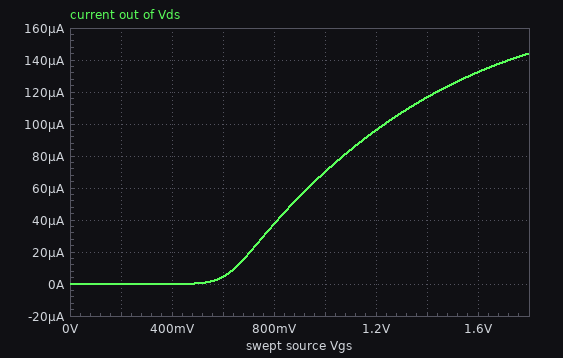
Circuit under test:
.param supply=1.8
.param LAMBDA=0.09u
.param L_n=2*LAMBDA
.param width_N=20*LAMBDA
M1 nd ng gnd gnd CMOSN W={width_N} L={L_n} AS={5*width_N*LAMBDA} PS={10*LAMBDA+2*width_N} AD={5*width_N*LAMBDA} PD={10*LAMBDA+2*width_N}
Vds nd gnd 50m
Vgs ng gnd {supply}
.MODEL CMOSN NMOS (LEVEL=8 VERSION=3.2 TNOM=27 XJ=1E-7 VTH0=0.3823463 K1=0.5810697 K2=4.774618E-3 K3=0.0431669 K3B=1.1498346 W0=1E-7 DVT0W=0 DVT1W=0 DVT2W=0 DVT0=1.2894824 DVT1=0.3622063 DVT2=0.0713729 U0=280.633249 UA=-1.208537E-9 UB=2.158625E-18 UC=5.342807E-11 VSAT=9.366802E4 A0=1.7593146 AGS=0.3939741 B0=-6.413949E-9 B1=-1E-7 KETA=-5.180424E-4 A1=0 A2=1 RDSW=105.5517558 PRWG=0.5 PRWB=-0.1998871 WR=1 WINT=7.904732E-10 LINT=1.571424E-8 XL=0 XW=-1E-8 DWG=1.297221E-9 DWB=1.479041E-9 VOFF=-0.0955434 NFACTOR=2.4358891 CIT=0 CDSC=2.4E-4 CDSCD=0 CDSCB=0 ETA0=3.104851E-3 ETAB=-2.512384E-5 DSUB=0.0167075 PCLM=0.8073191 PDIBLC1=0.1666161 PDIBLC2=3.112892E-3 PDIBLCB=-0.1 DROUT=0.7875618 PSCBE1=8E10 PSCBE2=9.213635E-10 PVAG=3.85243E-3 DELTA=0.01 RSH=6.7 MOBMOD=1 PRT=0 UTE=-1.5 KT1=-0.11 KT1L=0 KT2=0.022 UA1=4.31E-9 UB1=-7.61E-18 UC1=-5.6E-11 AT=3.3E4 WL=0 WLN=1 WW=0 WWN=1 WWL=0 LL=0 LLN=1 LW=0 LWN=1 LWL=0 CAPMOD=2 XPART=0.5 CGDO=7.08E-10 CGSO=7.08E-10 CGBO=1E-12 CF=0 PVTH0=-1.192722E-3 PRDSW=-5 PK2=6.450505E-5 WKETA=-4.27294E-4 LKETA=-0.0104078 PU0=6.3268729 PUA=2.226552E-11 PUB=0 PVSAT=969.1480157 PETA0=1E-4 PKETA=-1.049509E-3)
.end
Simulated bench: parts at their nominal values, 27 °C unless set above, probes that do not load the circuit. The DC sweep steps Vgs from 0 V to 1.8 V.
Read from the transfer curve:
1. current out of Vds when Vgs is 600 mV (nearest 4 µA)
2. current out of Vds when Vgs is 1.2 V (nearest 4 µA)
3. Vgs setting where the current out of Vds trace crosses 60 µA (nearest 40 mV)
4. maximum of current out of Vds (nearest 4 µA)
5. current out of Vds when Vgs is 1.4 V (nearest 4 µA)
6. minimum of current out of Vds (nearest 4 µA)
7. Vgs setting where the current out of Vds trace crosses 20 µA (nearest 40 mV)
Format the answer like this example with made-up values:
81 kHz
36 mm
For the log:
4 µA
96 µA
920 mV
144 µA
116 µA
0 A
720 mV
